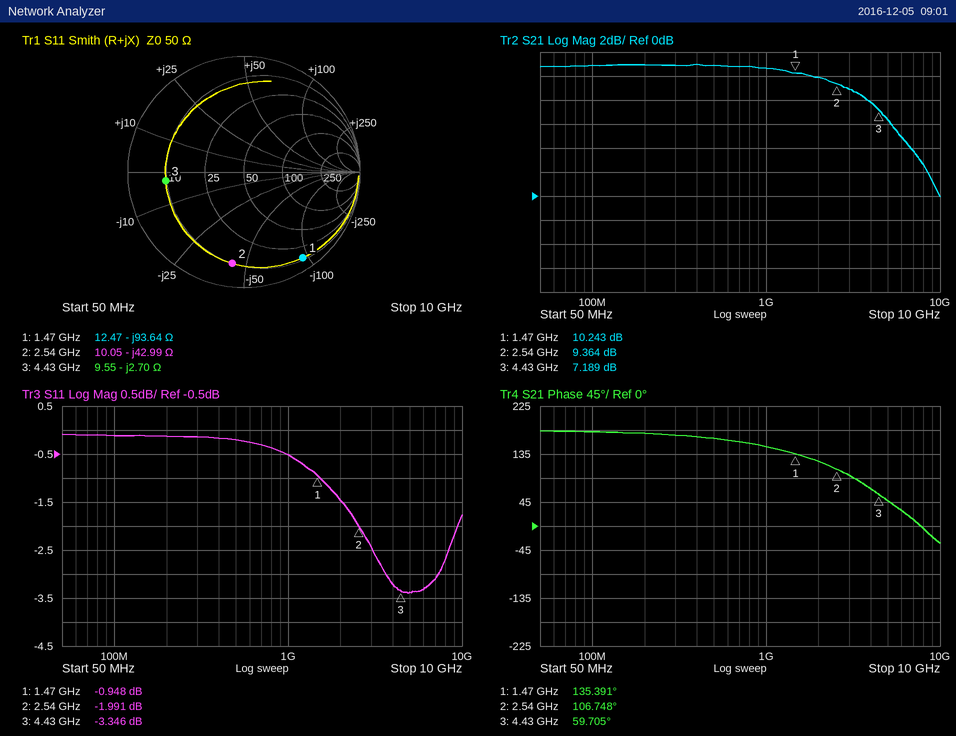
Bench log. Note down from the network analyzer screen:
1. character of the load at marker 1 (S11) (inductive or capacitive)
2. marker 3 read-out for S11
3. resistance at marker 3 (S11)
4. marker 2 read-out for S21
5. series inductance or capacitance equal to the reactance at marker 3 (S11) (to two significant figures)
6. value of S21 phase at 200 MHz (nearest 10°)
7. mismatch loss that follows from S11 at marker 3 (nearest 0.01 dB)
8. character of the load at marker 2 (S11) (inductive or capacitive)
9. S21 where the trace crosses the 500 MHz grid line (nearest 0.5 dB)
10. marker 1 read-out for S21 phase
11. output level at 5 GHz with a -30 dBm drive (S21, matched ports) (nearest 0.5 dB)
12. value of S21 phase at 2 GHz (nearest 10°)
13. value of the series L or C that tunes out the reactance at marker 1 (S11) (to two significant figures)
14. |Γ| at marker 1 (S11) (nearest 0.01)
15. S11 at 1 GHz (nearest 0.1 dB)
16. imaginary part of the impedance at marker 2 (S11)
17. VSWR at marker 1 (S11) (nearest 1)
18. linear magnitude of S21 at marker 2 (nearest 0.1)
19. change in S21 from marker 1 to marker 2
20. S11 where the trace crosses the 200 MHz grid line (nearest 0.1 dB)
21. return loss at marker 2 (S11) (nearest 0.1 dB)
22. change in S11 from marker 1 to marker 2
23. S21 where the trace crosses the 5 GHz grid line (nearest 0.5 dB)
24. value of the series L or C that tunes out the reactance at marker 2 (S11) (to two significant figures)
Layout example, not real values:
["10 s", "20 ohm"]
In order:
["capacitive", "-3.346 dB", "9.55 Ω", "9.364 dB", "13 pF", "170°", "2.70 dB", "capacitive", "11.0 dB", "135.391°", "-23.5 dBm", "120°", "10 nH", "0.90", "-0.5 dB", "-42.99 Ω", "18", "2.9", "-0.879 dB", "-0.1 dB", "2.0 dB", "-1.043 dB", "6.5 dB", "2.7 nH"]
